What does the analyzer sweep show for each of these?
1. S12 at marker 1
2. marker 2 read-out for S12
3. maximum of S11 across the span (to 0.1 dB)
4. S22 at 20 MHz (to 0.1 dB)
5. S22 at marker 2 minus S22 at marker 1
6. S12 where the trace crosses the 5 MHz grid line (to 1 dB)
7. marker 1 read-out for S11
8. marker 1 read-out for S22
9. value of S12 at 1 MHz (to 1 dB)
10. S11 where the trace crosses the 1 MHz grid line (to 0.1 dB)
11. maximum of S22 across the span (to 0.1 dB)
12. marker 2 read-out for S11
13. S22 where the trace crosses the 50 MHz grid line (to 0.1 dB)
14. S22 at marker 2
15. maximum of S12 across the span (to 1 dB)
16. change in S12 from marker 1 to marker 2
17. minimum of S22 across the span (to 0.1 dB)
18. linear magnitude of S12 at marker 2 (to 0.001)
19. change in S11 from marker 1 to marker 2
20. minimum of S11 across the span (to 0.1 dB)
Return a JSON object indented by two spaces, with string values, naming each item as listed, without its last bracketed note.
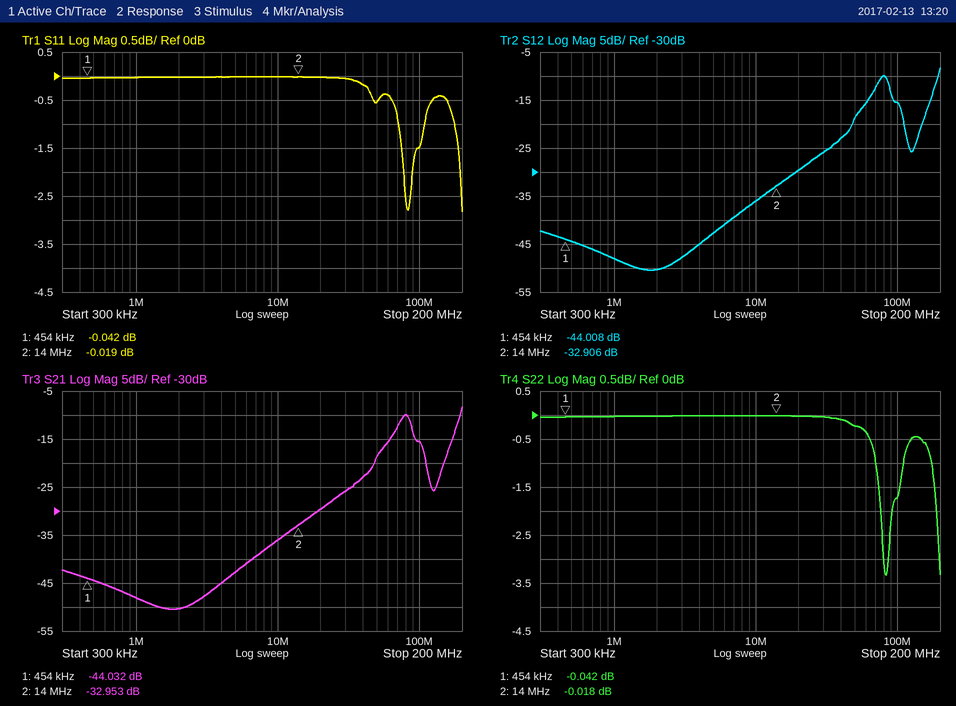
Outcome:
{
  "S12 at marker 1": "-44.008 dB",
  "marker 2 read-out for S12": "-32.906 dB",
  "maximum of S11 across the span": "0.0 dB",
  "S22 at 20 MHz": "0.0 dB",
  "S22 at marker 2 minus S22 at marker 1": "0.024 dB",
  "S12 where the trace crosses the 5 MHz grid line": "-43 dB",
  "marker 1 read-out for S11": "-0.042 dB",
  "marker 1 read-out for S22": "-0.042 dB",
  "value of S12 at 1 MHz": "-48 dB",
  "S11 where the trace crosses the 1 MHz grid line": "0.0 dB",
  "maximum of S22 across the span": "0.0 dB",
  "marker 2 read-out for S11": "-0.019 dB",
  "S22 where the trace crosses the 50 MHz grid line": "-0.2 dB",
  "S22 at marker 2": "-0.018 dB",
  "maximum of S12 across the span": "-8 dB",
  "change in S12 from marker 1 to marker 2": "11.102 dB",
  "minimum of S22 across the span": "-3.3 dB",
  "linear magnitude of S12 at marker 2": "0.023",
  "change in S11 from marker 1 to marker 2": "0.023 dB",
  "minimum of S11 across the span": "-2.8 dB"
}
